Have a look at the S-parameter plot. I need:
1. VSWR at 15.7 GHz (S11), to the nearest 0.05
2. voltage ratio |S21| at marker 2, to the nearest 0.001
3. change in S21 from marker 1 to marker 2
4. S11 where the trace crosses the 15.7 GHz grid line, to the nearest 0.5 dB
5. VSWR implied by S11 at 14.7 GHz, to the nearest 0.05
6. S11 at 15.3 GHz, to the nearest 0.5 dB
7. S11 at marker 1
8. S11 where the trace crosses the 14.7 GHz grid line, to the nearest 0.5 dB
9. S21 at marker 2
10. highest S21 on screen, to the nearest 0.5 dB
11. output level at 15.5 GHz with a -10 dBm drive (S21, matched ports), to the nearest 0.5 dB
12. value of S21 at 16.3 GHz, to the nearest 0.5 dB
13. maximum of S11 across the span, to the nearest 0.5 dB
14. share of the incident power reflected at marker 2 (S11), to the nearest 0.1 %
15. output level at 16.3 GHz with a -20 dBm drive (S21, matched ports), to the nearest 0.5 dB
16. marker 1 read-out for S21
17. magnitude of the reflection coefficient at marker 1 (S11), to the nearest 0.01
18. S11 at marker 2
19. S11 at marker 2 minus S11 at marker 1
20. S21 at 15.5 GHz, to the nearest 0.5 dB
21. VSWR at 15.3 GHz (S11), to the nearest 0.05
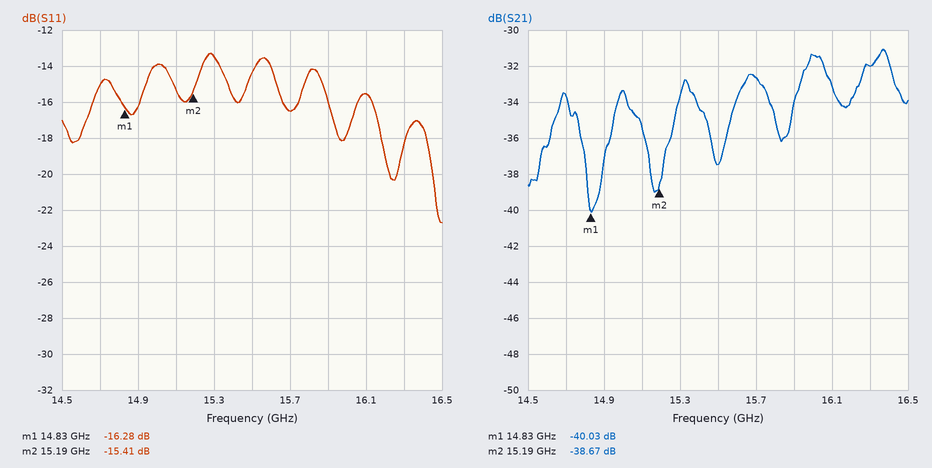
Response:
1.35
0.012
1.36 dB
-16.5 dB
1.45
-13.5 dB
-16.28 dB
-15.0 dB
-38.67 dB
-31.0 dB
-47.5 dBm
-32.0 dB
-13.5 dB
2.9 %
-52.0 dBm
-40.03 dB
0.15
-15.41 dB
0.87 dB
-37.5 dB
1.55
